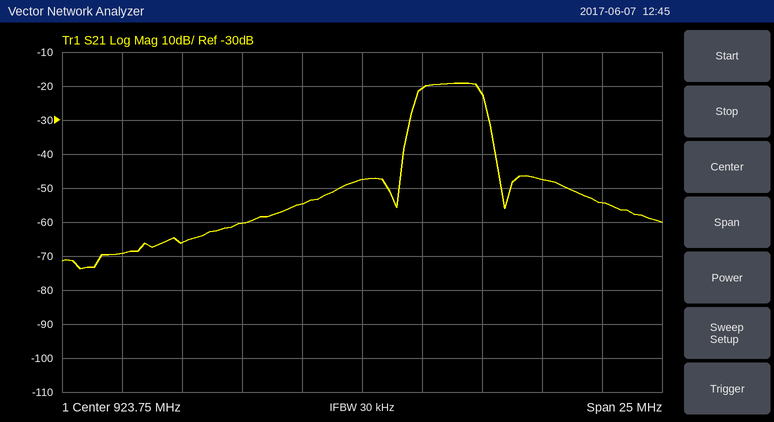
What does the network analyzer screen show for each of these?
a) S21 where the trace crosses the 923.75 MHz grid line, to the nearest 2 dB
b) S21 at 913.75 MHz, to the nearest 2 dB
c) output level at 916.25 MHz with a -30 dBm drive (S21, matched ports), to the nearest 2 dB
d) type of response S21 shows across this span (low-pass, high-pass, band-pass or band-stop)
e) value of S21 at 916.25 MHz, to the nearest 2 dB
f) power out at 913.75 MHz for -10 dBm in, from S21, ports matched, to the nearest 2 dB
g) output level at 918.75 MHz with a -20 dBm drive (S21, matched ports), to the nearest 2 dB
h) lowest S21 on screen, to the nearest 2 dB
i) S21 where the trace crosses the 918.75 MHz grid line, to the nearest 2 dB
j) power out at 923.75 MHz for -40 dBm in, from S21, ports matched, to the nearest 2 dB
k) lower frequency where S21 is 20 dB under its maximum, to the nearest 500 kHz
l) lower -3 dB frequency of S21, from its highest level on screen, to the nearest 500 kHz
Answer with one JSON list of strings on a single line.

["-48 dB", "-70 dB", "-96 dBm", "band-pass", "-66 dB", "-80 dBm", "-80 dBm", "-74 dB", "-60 dB", "-88 dBm", "925.5 MHz", "926.0 MHz"]
